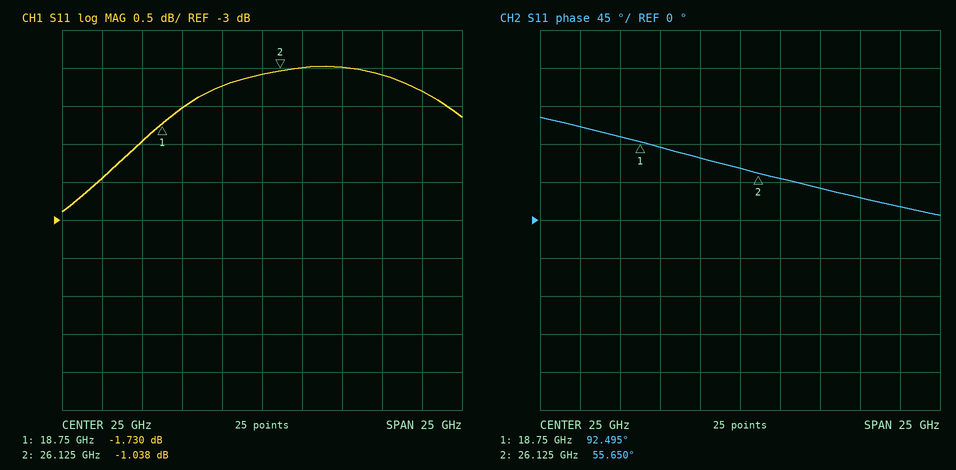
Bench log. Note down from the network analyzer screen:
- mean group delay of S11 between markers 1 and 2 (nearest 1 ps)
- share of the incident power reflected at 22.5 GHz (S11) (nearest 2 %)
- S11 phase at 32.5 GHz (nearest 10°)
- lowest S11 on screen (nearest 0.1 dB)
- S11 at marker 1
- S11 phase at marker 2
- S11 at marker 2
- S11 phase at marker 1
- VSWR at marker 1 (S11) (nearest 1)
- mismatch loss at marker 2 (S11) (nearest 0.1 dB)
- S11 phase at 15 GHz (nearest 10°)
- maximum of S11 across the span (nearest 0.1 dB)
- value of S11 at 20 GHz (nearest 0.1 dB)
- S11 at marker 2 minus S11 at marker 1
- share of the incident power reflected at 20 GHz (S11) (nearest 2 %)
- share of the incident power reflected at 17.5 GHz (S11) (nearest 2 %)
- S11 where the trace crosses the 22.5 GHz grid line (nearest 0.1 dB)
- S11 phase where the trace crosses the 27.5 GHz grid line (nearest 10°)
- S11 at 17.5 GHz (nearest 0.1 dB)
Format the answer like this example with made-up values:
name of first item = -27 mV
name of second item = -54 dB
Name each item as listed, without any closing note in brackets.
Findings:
mean group delay of S11 between markers 1 and 2 = 14 ps
share of the incident power reflected at 22.5 GHz (S11) = 76 %
S11 phase at 32.5 GHz = 30°
lowest S11 on screen = -2.9 dB
S11 at marker 1 = -1.730 dB
S11 phase at marker 2 = 55.650°
S11 at marker 2 = -1.038 dB
S11 phase at marker 1 = 92.495°
VSWR at marker 1 (S11) = 10
mismatch loss at marker 2 (S11) = 6.7 dB
S11 phase at 15 GHz = 110°
maximum of S11 across the span = -1.0 dB
value of S11 at 20 GHz = -1.5 dB
S11 at marker 2 minus S11 at marker 1 = 0.692 dB
share of the incident power reflected at 20 GHz (S11) = 70 %
share of the incident power reflected at 17.5 GHz (S11) = 64 %
S11 where the trace crosses the 22.5 GHz grid line = -1.2 dB
S11 phase where the trace crosses the 27.5 GHz grid line = 50°
S11 at 17.5 GHz = -2.0 dB
